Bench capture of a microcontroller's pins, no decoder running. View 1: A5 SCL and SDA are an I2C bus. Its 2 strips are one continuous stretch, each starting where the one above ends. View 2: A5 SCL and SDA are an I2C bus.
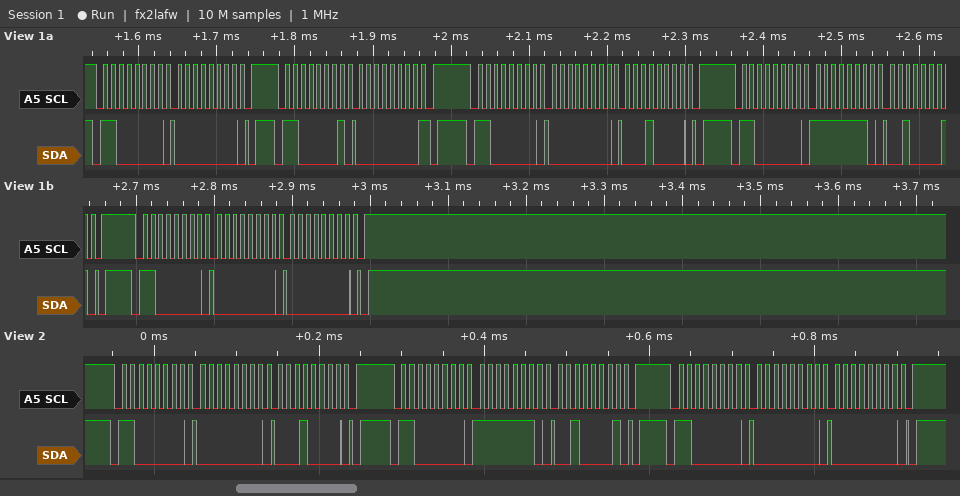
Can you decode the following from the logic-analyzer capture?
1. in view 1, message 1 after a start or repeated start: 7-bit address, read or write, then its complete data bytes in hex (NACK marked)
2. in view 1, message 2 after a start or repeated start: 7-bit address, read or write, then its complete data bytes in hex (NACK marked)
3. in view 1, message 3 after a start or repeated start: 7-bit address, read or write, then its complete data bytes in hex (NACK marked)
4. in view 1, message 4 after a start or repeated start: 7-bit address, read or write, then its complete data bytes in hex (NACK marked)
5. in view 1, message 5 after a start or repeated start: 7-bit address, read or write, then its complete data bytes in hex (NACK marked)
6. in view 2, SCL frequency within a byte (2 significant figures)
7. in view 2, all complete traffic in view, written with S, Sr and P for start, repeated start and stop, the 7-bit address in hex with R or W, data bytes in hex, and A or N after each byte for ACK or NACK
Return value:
0x60 write: 00
0x60 read: 00 NACK
0x60 write: 00 10
0x60 write: FE 21
0x60 write: 00 00
100 kHz
S 60W A 00 A 10 A P S 60W A FE A 21 A P S 60W A 00 A 00 A P
